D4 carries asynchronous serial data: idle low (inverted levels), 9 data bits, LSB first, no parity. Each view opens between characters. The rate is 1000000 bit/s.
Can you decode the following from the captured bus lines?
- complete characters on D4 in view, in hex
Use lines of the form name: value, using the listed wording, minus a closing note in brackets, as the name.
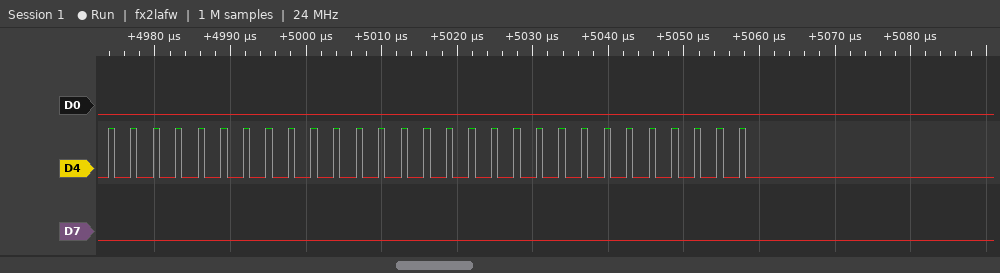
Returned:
complete characters on D4 in view, in hex: DB, DB, DB, DB, DB, DB, DB, 1FF
